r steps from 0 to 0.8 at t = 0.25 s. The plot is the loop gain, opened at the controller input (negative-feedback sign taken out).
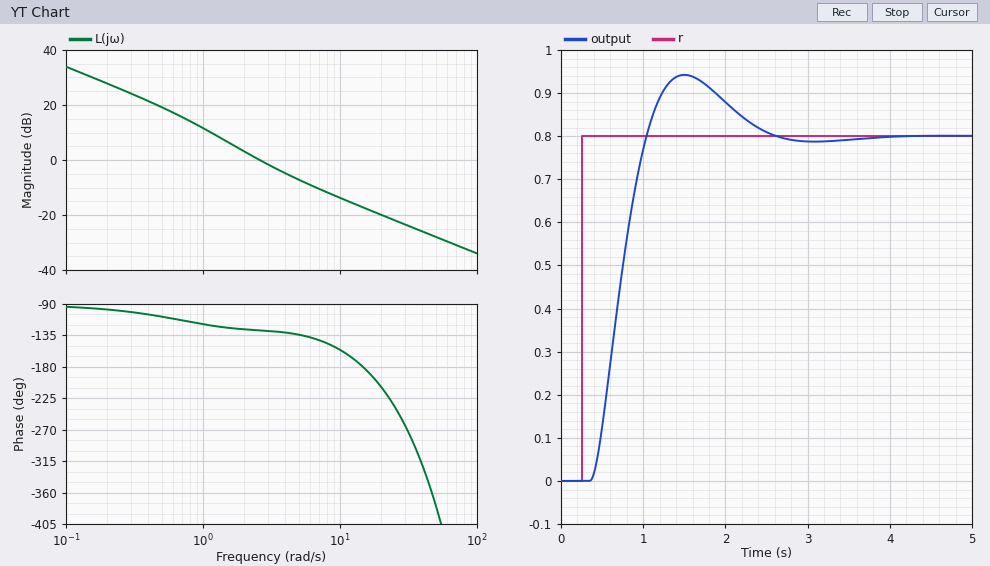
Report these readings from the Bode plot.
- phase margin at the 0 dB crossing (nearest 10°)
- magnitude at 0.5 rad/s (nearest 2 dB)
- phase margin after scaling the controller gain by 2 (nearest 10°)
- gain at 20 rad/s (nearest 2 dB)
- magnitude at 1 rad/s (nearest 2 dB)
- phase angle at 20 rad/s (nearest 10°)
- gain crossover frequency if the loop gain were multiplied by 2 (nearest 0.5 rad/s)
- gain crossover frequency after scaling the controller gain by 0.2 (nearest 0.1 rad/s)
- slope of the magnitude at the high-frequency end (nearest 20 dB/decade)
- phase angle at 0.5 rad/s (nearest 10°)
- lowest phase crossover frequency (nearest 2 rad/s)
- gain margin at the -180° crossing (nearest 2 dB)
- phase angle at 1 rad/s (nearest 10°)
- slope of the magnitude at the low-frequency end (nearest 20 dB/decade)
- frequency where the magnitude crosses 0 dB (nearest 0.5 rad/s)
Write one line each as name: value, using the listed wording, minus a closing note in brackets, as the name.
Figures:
phase margin at the 0 dB crossing: 50°
magnitude at 0.5 rad/s: 20 dB
phase margin after scaling the controller gain by 2: 50°
gain at 20 rad/s: -20 dB
magnitude at 1 rad/s: 12 dB
phase angle at 20 rad/s: -210°
gain crossover frequency if the loop gain were multiplied by 2: 4.5 rad/s
gain crossover frequency after scaling the controller gain by 0.2: 0.8 rad/s
slope of the magnitude at the high-frequency end: -20 dB/decade
phase angle at 0.5 rad/s: -110°
lowest phase crossover frequency: 14 rad/s
gain margin at the -180° crossing: 18 dB
phase angle at 1 rad/s: -120°
slope of the magnitude at the low-frequency end: -20 dB/decade
frequency where the magnitude crosses 0 dB: 2.5 rad/s
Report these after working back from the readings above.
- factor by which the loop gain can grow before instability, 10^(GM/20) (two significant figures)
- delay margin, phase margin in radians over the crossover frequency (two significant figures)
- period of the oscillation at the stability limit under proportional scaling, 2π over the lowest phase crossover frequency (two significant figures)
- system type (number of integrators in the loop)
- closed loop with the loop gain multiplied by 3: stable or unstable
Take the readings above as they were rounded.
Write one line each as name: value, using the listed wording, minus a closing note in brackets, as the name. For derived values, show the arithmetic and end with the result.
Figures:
factor by which the loop gain can grow before instability, 10^(GM/20): 10^(18 / 20) = 7.9
delay margin, phase margin in radians over the crossover frequency: 50 × π / 180 / 2.5 = 0.35 s
period of the oscillation at the stability limit under proportional scaling, 2π over the lowest phase crossover frequency: 2π / 14 = 0.45 s
system type: 1
closed loop with the loop gain multiplied by 3: stable or unstable: stable
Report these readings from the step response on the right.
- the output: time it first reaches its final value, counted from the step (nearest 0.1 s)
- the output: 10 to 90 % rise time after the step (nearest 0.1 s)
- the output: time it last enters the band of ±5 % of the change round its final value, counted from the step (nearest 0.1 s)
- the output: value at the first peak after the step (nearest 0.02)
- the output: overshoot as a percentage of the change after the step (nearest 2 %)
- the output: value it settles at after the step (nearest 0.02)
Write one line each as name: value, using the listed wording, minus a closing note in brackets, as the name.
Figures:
the output: time it first reaches its final value, counted from the step: 0.8 s
the output: 10 to 90 % rise time after the step: 0.5 s
the output: time it last enters the band of ±5 % of the change round its final value, counted from the step: 2.0 s
the output: value at the first peak after the step: 0.94
the output: overshoot as a percentage of the change after the step: 18 %
the output: value it settles at after the step: 0.80
